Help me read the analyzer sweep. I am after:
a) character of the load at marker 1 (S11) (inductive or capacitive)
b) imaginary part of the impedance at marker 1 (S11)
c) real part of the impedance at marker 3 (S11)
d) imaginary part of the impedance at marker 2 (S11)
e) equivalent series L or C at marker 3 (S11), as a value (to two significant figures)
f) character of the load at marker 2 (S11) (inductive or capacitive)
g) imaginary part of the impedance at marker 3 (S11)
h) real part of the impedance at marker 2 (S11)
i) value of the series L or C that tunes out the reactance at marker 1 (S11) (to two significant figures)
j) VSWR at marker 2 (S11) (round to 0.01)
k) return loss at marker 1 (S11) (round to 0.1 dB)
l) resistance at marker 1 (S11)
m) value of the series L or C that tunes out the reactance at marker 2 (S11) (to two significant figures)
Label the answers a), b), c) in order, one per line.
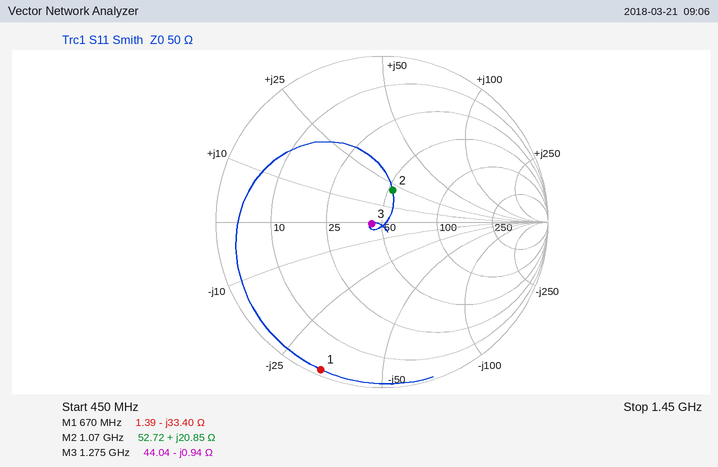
a) capacitive
b) -33.40 Ω
c) 44.04 Ω
d) +20.85 Ω
e) 130 pF
f) inductive
g) -0.94 Ω
h) 52.72 Ω
i) 7.9 nH
j) 1.50
k) 0.3 dB
l) 1.39 Ω
m) 7.1 pF
